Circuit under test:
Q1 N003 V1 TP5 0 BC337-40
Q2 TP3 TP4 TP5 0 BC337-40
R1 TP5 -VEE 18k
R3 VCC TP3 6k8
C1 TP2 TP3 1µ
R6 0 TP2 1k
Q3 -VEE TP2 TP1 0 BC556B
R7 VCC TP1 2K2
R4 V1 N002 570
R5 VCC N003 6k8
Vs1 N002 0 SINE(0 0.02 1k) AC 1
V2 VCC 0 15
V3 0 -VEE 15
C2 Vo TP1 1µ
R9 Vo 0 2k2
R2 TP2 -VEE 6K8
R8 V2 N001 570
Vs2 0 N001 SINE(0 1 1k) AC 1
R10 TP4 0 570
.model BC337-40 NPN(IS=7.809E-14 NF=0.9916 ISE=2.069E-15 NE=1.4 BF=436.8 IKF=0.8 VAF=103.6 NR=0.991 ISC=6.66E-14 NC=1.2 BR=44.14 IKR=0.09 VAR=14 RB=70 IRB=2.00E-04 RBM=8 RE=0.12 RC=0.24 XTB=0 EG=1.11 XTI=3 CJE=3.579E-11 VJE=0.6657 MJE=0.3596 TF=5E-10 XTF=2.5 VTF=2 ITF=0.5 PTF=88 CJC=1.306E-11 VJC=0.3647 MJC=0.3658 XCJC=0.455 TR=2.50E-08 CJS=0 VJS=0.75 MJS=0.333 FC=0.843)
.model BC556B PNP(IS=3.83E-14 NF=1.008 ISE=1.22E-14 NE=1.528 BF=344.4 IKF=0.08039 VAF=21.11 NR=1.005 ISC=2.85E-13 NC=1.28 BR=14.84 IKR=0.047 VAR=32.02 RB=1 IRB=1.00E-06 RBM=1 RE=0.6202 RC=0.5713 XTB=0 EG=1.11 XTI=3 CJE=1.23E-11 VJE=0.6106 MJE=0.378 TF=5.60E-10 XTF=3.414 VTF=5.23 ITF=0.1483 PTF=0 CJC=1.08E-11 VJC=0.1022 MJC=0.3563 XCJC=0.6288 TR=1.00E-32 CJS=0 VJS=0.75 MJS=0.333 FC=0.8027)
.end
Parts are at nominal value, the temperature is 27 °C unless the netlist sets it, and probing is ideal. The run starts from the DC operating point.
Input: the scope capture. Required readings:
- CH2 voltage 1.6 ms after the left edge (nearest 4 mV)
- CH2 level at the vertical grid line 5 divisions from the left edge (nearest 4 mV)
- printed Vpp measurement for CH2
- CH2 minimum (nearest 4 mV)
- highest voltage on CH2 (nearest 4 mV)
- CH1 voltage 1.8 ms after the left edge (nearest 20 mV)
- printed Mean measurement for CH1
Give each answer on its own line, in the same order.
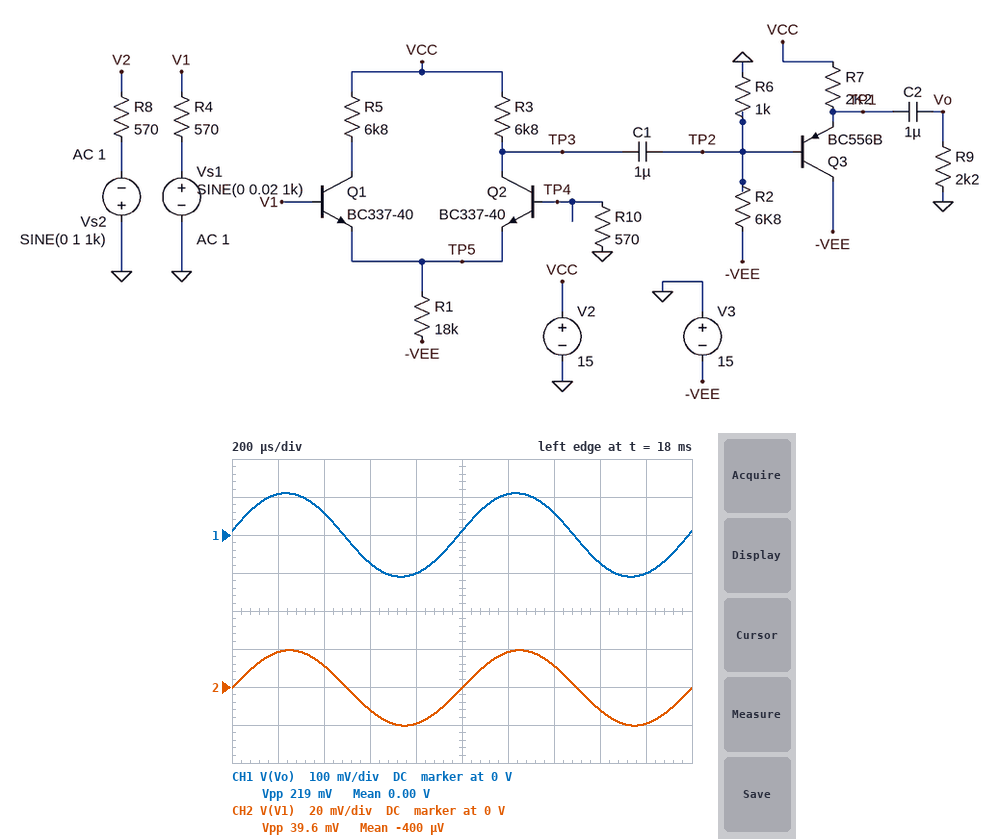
-12 mV
0 V
39.6 mV
-20 mV
20 mV
-100 mV
0.00 V
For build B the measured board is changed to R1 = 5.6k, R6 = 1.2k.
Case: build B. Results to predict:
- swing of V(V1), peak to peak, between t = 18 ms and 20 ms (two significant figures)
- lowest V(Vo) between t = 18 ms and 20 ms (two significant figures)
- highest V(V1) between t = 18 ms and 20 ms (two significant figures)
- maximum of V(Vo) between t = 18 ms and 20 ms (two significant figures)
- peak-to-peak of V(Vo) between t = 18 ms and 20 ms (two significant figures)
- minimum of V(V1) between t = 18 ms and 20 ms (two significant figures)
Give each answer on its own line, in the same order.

39 mV
-370 mV
18 mV
370 mV
750 mV
-21 mV
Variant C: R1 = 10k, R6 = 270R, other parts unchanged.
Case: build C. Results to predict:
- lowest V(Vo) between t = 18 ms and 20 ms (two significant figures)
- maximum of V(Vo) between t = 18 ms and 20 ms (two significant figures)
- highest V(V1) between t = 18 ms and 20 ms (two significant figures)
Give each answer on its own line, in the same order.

-62 mV
62 mV
19 mV
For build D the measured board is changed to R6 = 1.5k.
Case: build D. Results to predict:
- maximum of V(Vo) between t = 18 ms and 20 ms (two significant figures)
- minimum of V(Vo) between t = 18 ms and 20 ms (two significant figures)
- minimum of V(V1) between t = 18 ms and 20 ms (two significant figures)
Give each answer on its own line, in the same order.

150 mV
-150 mV
-20 mV
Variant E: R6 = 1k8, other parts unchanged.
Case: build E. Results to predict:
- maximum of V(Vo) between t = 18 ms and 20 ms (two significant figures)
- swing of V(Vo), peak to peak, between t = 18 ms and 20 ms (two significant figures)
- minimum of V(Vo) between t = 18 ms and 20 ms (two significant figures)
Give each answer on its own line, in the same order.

170 mV
330 mV
-170 mV
